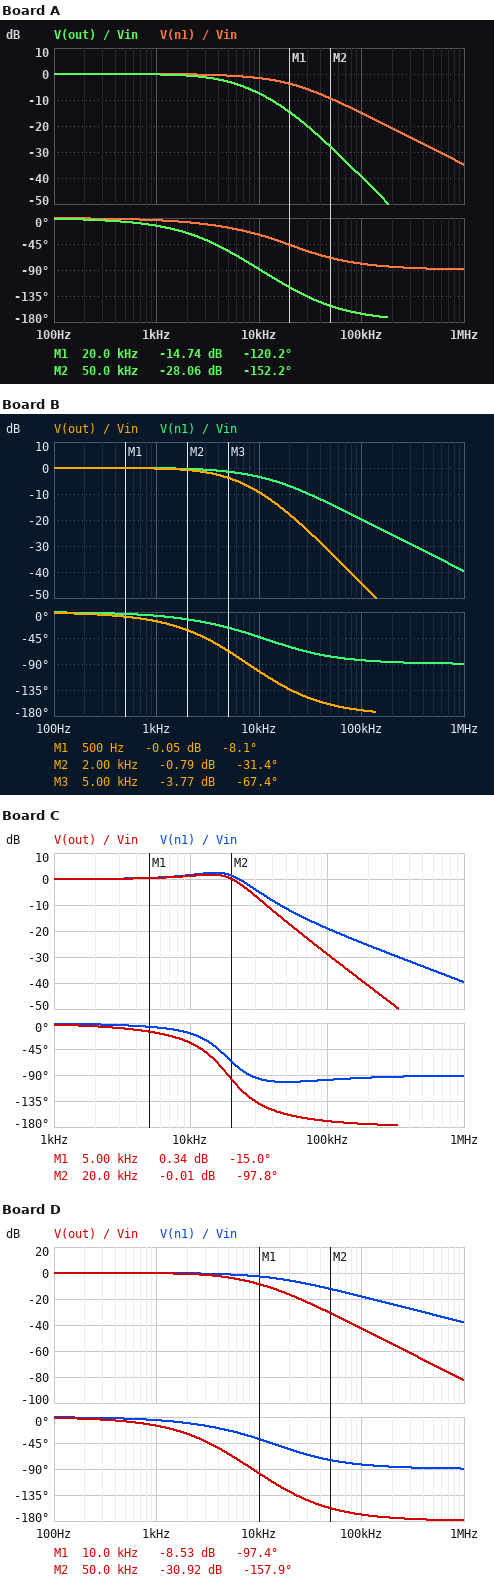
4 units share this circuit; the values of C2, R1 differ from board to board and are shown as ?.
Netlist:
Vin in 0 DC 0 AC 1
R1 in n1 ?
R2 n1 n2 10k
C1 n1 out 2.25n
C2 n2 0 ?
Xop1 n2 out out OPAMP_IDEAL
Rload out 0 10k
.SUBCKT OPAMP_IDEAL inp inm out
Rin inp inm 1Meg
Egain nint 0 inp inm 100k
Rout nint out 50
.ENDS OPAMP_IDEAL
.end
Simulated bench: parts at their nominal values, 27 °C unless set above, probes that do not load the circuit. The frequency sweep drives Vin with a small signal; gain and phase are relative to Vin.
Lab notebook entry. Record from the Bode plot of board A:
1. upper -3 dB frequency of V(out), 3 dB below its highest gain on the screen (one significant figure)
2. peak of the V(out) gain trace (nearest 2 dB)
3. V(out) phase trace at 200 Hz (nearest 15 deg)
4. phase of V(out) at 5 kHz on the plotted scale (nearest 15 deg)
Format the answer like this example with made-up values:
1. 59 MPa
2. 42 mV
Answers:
1. 5 kHz
2. 0 dB
3. 0 deg
4. -60 deg
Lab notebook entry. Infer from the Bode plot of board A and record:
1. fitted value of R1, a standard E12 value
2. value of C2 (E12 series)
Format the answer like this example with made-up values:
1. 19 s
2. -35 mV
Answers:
1. 3.9 kΩ
2. 2.7 nF
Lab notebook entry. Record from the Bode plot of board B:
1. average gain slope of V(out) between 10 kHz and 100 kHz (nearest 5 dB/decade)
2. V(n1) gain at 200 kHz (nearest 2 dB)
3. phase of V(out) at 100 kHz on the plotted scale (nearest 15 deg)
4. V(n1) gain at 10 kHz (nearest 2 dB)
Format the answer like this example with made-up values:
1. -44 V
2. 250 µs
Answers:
1. -35 dB/decade
2. -26 dB
3. -165 deg
4. -4 dB
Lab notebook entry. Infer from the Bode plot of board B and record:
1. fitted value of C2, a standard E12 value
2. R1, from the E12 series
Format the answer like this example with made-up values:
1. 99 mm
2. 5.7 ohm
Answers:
1. 2.7 nF
2. 6.8 kΩ
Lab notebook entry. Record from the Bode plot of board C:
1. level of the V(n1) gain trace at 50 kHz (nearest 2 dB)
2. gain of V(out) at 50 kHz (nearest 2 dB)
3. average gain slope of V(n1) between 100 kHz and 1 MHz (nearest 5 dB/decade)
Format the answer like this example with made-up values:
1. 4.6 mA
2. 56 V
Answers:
1. -12 dB
2. -16 dB
3. -20 dB/decade
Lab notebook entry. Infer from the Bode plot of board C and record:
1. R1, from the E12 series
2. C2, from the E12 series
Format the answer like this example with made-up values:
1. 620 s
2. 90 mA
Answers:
1. 6.8 kΩ
2. 470 pF
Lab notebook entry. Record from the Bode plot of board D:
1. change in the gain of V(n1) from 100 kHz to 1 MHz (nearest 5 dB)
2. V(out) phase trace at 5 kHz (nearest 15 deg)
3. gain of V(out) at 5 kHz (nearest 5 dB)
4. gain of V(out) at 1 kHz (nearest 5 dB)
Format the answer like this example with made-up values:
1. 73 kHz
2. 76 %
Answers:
1. -20 dB
2. -60 deg
3. -5 dB
4. 0 dB
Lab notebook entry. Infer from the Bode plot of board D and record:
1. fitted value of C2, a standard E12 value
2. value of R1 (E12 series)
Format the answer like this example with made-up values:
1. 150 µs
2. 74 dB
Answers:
1. 2.7 nF
2. 5.6 kΩ
